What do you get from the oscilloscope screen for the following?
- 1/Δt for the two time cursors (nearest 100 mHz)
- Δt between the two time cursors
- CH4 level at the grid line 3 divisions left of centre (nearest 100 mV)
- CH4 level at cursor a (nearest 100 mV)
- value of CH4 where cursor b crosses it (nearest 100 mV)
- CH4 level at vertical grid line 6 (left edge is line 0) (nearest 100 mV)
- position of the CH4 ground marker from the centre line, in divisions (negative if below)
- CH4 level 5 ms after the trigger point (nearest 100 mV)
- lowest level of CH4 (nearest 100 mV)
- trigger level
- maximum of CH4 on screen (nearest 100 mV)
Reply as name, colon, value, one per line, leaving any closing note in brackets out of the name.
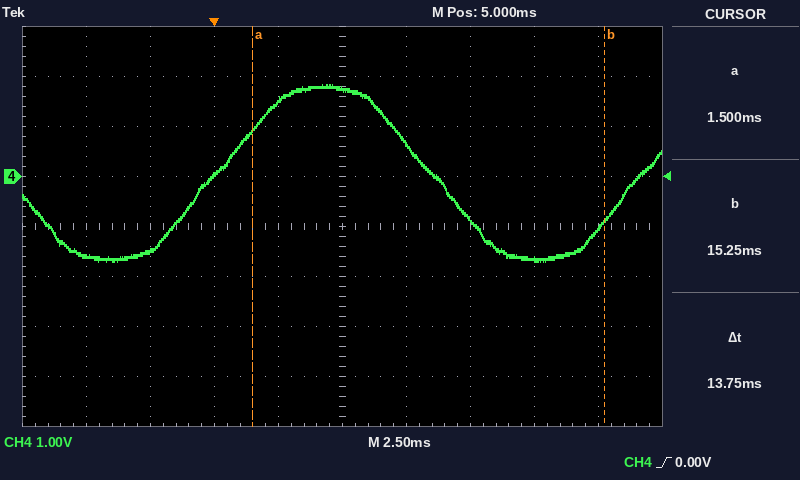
1/Δt for the two time cursors: 72.7 Hz
Δt between the two time cursors: 13.75 ms
CH4 level at the grid line 3 divisions left of centre: -1.5 V
CH4 level at cursor a: 900 mV
value of CH4 where cursor b crosses it: -900 mV
CH4 level at vertical grid line 6 (left edge is line 0): 700 mV
position of the CH4 ground marker from the centre line, in divisions: +1.0 div
CH4 level 5 ms after the trigger point: 1.7 V
lowest level of CH4: -1.7 V
trigger level: 0.00 V
maximum of CH4 on screen: 1.8 V
